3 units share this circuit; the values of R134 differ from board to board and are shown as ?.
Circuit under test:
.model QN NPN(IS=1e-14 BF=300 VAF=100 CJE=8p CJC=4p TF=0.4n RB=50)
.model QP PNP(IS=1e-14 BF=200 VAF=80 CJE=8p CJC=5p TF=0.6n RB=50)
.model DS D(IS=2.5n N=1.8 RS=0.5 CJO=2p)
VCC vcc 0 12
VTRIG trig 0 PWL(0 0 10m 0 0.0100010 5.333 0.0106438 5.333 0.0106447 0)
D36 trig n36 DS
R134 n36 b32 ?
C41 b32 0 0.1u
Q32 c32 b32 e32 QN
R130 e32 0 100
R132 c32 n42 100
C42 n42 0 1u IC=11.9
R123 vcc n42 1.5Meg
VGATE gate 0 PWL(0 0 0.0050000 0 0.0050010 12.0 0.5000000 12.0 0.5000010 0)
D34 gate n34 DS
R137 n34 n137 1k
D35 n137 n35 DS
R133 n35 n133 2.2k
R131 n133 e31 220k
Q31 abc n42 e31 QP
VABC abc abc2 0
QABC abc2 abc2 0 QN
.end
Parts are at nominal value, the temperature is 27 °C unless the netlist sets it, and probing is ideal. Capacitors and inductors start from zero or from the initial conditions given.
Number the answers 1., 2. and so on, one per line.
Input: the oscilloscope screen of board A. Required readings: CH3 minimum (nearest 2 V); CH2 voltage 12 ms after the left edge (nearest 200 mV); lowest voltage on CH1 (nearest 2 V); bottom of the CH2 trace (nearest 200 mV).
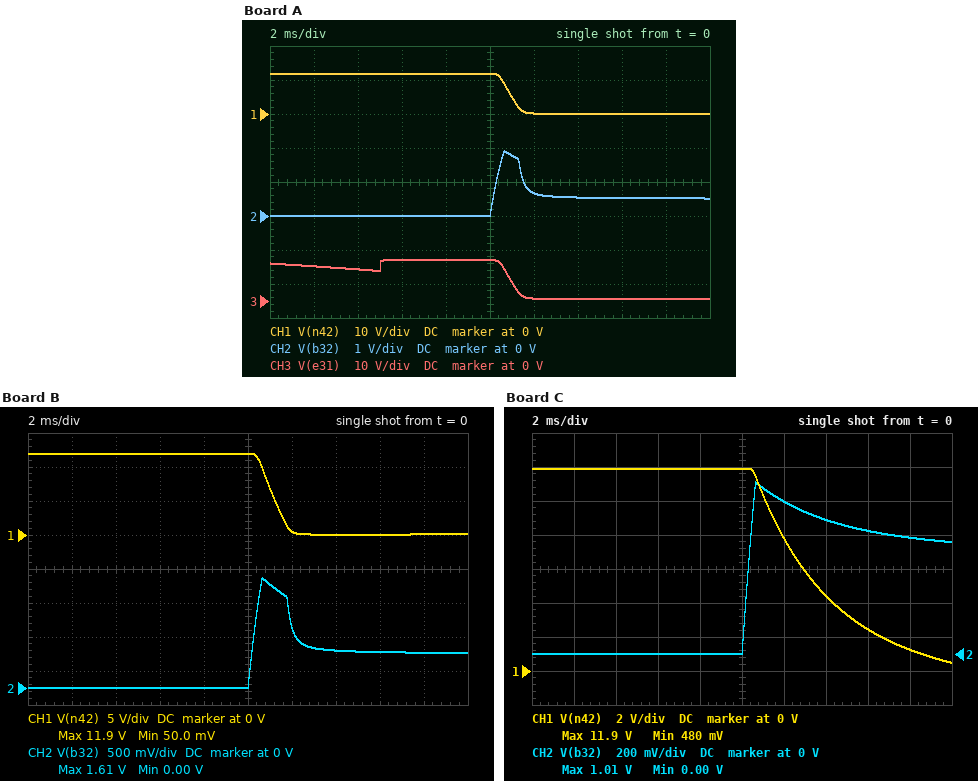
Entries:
1. 0 V
2. 600 mV
3. 0 V
4. 0 V
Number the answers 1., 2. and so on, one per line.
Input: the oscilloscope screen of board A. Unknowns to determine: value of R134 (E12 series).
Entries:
1. 12 kΩ
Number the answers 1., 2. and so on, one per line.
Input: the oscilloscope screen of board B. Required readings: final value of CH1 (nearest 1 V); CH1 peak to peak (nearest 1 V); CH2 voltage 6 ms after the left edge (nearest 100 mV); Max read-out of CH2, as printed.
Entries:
1. 0 V
2. 12 V
3. 0 V
4. 1.61 V
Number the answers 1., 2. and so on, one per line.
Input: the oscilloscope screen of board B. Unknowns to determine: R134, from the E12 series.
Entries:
1. 15 kΩ
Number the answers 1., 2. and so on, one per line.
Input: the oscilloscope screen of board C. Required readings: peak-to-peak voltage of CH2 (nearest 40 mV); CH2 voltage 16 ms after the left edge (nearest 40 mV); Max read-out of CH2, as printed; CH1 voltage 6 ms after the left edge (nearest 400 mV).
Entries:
1. 1.00 V
2. 720 mV
3. 1.01 V
4. 12.0 V
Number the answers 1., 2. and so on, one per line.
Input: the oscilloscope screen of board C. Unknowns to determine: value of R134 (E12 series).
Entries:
1. 27 kΩ
